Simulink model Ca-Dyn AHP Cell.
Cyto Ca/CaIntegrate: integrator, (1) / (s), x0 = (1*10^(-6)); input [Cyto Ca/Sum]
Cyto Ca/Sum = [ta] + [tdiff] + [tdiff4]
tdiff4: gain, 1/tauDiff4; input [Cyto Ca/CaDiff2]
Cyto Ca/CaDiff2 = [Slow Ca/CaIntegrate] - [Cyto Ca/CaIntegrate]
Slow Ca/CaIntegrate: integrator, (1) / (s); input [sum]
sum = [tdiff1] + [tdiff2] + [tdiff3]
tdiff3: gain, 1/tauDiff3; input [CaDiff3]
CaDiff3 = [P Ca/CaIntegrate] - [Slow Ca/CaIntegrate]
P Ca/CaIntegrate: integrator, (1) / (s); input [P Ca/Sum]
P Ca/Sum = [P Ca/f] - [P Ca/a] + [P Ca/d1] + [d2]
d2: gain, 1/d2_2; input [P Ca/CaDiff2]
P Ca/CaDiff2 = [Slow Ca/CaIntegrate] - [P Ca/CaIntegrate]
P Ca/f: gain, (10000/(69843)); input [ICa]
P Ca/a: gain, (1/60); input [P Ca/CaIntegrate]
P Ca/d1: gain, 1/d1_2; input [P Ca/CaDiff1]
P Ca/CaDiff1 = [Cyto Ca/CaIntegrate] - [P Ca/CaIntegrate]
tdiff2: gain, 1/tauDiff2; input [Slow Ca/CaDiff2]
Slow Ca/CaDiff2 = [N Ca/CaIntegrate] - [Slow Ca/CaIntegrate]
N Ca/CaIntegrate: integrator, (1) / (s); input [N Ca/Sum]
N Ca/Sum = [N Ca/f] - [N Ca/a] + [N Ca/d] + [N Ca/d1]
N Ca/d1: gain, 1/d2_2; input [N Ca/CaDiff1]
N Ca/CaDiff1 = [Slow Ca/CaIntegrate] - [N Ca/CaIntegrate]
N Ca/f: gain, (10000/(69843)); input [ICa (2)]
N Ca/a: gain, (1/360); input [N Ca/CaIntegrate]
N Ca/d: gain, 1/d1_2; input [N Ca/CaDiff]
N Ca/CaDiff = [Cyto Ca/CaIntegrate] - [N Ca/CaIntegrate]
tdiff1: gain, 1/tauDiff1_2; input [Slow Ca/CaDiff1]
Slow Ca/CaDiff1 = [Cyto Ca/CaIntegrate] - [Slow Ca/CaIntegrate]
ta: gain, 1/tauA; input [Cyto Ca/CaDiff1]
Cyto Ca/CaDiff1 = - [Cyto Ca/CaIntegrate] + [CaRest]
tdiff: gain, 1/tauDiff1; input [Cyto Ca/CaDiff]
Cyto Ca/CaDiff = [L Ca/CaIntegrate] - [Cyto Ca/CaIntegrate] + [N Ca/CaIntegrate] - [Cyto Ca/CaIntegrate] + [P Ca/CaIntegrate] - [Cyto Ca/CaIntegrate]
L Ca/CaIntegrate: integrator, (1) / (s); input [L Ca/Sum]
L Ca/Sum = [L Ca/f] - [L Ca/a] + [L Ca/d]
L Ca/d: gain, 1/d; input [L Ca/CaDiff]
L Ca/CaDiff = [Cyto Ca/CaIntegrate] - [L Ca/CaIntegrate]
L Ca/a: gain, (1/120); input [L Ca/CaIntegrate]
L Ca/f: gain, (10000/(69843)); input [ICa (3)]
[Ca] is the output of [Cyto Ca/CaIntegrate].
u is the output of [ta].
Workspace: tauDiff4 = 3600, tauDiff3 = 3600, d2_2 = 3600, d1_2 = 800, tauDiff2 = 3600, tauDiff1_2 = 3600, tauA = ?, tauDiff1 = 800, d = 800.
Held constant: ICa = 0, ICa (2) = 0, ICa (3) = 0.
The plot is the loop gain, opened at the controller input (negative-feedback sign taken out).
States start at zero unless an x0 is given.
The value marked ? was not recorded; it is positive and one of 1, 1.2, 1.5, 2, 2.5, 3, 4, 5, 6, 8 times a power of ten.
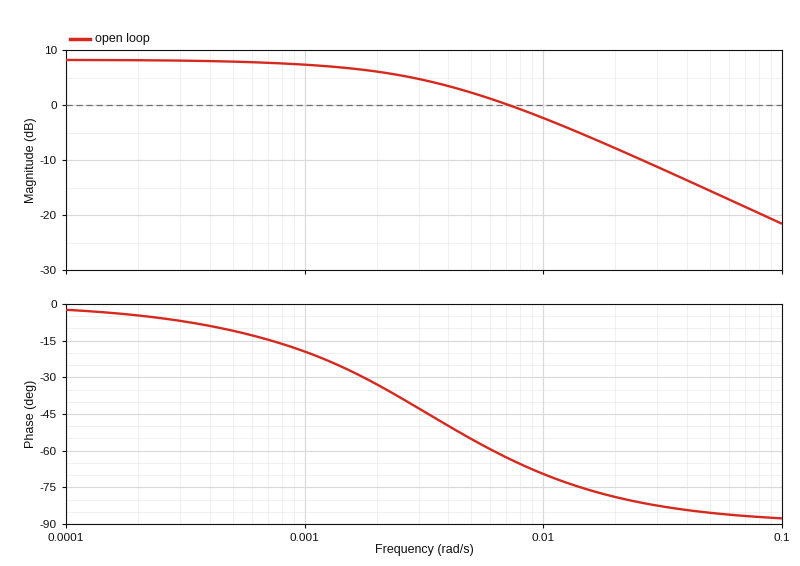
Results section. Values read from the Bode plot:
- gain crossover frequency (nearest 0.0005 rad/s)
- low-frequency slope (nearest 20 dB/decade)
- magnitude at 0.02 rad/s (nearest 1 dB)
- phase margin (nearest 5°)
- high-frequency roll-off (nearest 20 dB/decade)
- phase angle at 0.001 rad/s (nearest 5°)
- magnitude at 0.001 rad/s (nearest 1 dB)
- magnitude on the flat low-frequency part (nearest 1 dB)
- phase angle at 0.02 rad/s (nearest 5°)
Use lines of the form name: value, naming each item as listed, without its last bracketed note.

gain crossover frequency: 0.0070 rad/s
low-frequency slope: 0 dB/decade
magnitude at 0.02 rad/s: -8 dB
phase margin: 115°
high-frequency roll-off: -20 dB/decade
phase angle at 0.001 rad/s: -20°
magnitude at 0.001 rad/s: 7 dB
magnitude on the flat low-frequency part: 8 dB
phase angle at 0.02 rad/s: -80°
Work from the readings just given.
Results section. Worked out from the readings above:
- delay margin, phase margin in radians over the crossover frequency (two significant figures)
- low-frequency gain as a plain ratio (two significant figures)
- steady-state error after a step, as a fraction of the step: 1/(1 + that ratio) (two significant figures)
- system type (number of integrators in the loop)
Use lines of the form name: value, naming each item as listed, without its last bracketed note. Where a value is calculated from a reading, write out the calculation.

delay margin, phase margin in radians over the crossover frequency: 115 × π / 180 / 0.007 = 290 s
low-frequency gain as a plain ratio: 10^(8 / 20) = 2.5
steady-state error after a step, as a fraction of the step: 1/(1 + that ratio): 1 / (1 + 2.5) = 0.29
system type: 0
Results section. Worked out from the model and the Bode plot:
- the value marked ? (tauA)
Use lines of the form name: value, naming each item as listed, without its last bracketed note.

the value marked ?: 120
